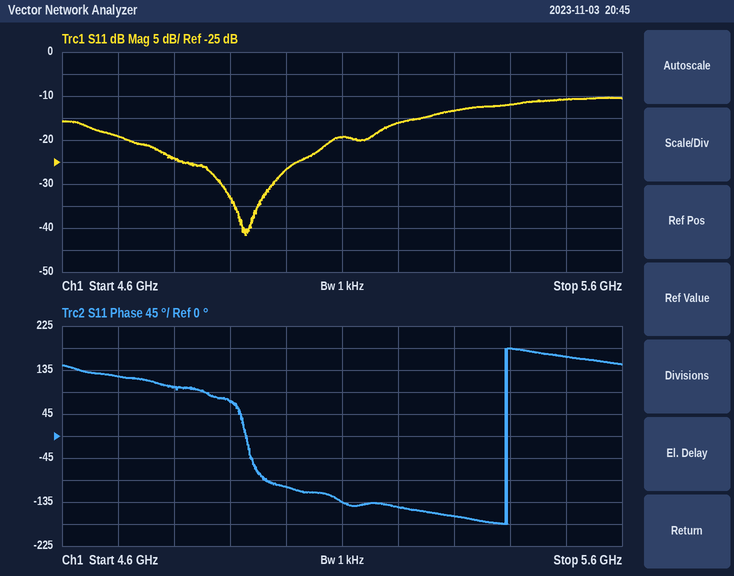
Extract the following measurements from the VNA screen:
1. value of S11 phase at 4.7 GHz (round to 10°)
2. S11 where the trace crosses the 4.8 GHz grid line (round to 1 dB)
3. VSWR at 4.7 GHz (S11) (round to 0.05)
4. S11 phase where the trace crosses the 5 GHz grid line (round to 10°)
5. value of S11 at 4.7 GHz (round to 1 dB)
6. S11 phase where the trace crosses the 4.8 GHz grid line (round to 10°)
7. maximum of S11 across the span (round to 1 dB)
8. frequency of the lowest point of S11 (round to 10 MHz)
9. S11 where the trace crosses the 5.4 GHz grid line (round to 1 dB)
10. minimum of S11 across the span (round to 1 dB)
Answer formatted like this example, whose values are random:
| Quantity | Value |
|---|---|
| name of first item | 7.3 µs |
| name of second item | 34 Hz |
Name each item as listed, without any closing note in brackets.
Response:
| Quantity | Value |
|---|---|
| value of S11 phase at 4.7 GHz | 120° |
| S11 where the trace crosses the 4.8 GHz grid line | -24 dB |
| VSWR at 4.7 GHz (S11) | 1.25 |
| S11 phase where the trace crosses the 5 GHz grid line | -100° |
| value of S11 at 4.7 GHz | -19 dB |
| S11 phase where the trace crosses the 4.8 GHz grid line | 100° |
| maximum of S11 across the span | -10 dB |
| frequency of the lowest point of S11 | 4.93 GHz |
| S11 where the trace crosses the 5.4 GHz grid line | -12 dB |
| minimum of S11 across the span | -42 dB |
